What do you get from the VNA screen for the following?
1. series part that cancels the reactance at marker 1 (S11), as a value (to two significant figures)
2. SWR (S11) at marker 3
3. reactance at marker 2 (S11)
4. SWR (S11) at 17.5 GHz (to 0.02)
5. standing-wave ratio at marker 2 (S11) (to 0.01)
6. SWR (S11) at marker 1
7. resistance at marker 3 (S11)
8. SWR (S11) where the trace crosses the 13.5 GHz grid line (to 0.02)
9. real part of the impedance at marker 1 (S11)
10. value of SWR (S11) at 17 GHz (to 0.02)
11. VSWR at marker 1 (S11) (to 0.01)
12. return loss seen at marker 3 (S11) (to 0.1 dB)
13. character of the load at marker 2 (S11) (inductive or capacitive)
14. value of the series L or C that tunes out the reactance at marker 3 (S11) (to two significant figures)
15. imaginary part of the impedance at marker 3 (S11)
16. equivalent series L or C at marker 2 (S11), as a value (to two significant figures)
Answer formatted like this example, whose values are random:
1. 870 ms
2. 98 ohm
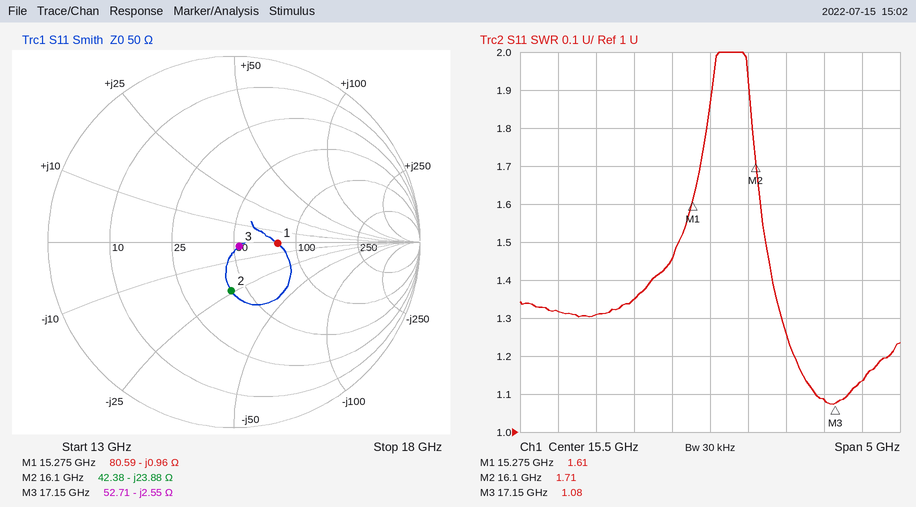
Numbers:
1. 10.0 pH
2. 1.08
3. -23.88 Ω
4. 1.14
5. 1.71
6. 1.61
7. 52.71 Ω
8. 1.32
9. 80.59 Ω
10. 1.08
11. 1.61
12. 28.8 dB
13. capacitive
14. 24 pH
15. -2.55 Ω
16. 410 fF
